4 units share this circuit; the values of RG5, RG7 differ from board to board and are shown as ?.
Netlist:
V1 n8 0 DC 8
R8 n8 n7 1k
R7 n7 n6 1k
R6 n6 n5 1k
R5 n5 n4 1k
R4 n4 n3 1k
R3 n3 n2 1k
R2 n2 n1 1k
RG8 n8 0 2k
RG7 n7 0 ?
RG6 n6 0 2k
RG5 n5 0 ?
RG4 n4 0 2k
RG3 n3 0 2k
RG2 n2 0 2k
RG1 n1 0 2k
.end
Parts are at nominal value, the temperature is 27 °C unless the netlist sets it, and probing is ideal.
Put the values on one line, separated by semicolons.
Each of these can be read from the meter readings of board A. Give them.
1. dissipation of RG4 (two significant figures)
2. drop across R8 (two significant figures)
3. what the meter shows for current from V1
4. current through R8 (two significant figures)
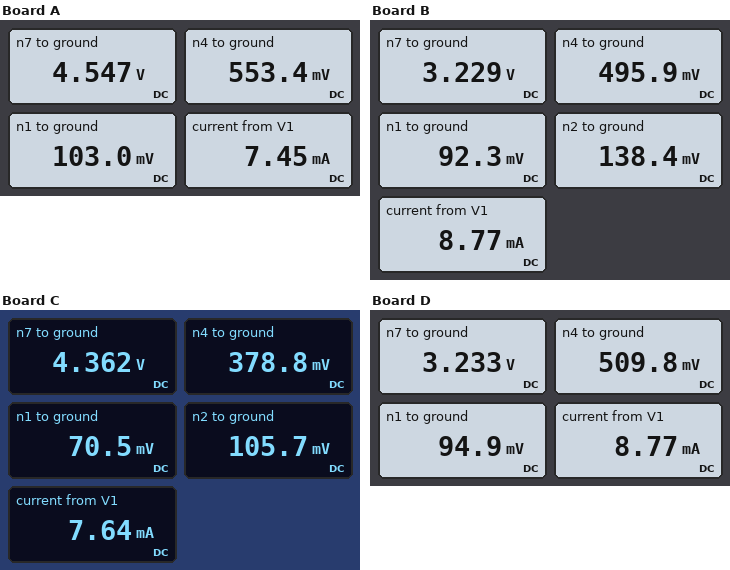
150 µW; 3.5 V; 7.45 mA; 3.5 mA
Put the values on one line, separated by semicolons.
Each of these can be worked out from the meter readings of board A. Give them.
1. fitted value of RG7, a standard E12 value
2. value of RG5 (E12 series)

3.9 kΩ; 1.8 kΩ
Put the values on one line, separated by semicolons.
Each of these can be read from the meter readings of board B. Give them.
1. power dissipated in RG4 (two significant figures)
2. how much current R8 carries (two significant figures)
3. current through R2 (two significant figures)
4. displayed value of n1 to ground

120 µW; 4.8 mA; 46 µA; 92.3 mV
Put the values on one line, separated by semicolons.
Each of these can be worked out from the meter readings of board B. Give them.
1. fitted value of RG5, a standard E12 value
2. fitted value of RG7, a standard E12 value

4.7 kΩ; 1 kΩ
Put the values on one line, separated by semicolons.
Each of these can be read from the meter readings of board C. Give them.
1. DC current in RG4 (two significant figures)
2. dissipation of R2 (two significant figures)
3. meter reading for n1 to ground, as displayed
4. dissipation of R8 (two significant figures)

190 µA; 1.2 µW; 70.5 mV; 13 mW
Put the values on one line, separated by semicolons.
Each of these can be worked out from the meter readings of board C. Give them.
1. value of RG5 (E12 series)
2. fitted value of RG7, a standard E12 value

820 Ω; 3.3 kΩ
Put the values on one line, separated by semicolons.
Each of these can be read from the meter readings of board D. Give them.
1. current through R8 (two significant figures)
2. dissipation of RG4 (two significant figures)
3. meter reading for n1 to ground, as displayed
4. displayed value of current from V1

4.8 mA; 130 µW; 94.9 mV; 8.77 mA
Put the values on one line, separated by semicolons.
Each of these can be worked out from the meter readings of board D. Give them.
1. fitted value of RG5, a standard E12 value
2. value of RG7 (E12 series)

5.6 kΩ; 1 kΩ
